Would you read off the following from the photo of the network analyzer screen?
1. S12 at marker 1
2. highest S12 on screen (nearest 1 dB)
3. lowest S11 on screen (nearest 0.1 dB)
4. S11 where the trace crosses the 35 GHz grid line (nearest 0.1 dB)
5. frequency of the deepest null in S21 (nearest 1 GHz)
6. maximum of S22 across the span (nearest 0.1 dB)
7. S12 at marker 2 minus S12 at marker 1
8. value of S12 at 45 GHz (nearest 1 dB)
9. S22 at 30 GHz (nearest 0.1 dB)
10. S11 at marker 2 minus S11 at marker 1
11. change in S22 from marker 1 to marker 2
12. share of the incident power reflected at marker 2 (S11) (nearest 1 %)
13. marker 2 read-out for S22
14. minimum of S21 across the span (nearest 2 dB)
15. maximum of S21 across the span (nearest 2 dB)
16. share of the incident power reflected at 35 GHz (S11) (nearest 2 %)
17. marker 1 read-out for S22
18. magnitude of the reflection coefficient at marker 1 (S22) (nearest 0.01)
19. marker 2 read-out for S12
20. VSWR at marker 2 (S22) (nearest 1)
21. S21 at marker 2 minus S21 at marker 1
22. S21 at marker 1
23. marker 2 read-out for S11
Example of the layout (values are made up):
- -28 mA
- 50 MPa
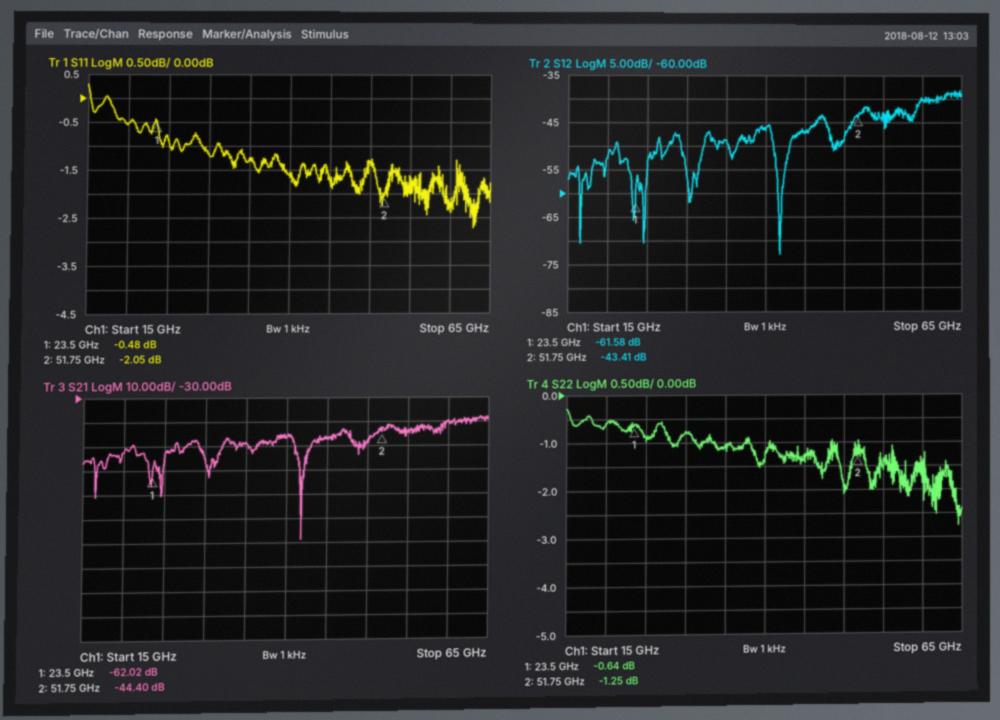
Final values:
- -61.58 dB
- -38 dB
- -2.7 dB
- -1.3 dB
- 42 GHz
- -0.3 dB
- 18.17 dB
- -47 dB
- -0.8 dB
- -1.57 dB
- -0.61 dB
- 62 %
- -1.25 dB
- -88 dB
- -38 dB
- 74 %
- -0.64 dB
- 0.93
- -43.41 dB
- 14
- 17.62 dB
- -62.02 dB
- -2.05 dB
